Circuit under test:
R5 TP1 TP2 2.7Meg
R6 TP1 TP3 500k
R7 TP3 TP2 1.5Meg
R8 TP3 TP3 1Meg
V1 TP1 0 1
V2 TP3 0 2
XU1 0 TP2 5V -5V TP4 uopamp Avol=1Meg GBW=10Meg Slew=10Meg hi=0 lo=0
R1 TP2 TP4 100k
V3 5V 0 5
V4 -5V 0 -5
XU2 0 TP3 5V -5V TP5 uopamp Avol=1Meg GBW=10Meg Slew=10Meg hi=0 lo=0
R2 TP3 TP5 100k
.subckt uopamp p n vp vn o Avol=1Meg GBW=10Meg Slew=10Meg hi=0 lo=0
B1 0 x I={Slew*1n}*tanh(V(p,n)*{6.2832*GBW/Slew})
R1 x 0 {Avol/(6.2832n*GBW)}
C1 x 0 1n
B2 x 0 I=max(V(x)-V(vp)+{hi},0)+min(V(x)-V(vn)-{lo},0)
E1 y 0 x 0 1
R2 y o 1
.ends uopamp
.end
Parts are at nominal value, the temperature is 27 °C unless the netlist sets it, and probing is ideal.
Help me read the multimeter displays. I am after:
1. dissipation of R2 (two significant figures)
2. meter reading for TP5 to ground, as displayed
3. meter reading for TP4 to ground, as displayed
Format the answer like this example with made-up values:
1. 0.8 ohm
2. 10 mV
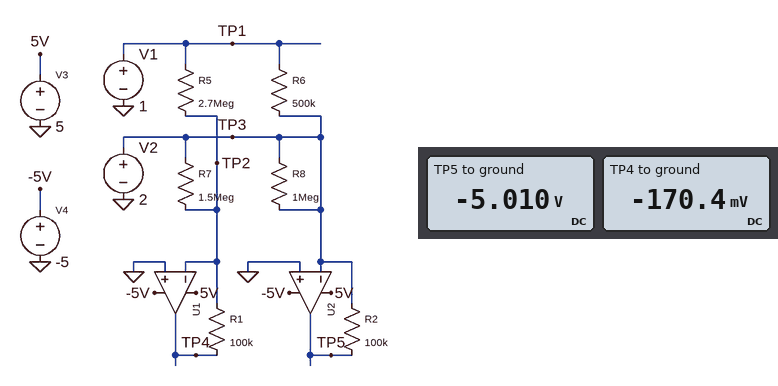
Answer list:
1. 490 µW
2. -5.010 V
3. -170.4 mV
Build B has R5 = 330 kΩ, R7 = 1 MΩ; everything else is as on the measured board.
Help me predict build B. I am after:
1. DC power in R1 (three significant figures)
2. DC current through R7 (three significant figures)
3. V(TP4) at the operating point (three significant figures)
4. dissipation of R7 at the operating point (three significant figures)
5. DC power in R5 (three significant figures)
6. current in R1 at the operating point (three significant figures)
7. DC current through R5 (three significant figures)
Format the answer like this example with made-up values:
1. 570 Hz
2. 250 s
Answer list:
1. 2.53 µW
2. 2.00 µA
3. -503 mV
4. 4.00 µW
5. 3.03 µW
6. 5.03 µA
7. 3.03 µA
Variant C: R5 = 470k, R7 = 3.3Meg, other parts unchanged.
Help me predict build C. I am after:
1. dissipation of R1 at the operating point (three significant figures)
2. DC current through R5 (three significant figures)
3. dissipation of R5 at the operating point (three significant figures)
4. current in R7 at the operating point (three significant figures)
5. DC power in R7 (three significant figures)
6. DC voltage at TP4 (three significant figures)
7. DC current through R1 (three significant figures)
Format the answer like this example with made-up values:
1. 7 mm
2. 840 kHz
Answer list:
1. 747 nW
2. 2.13 µA
3. 2.13 µW
4. 606 nA
5. 1.21 µW
6. -273 mV
7. 2.73 µA
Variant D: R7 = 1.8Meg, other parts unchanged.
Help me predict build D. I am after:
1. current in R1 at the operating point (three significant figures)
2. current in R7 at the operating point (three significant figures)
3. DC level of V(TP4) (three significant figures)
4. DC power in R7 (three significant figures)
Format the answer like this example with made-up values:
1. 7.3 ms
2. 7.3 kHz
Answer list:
1. 1.48 µA
2. 1.11 µA
3. -148 mV
4. 2.22 µW
